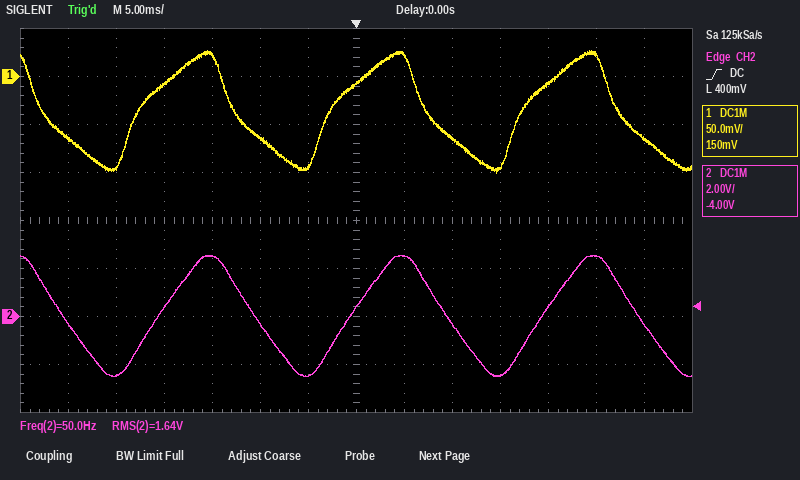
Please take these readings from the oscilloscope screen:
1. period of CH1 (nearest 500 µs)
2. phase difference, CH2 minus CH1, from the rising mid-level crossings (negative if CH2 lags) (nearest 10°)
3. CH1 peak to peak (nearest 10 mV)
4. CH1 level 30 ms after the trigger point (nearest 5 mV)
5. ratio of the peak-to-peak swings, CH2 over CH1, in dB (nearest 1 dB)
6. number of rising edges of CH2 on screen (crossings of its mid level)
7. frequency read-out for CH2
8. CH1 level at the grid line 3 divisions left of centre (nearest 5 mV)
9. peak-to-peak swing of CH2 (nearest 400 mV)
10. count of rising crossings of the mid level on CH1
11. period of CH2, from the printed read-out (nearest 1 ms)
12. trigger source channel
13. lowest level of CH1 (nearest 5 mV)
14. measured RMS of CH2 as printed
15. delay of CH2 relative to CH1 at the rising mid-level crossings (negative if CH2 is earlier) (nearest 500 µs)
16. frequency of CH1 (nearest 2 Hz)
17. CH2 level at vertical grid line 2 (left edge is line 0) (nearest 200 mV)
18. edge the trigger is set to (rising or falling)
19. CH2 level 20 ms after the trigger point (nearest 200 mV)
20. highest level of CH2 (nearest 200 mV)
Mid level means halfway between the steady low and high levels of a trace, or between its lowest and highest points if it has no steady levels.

20.0 ms
-40°
130 mV
-65 mV
32 dB
3
50.0 Hz
20 mV
5.2 V
3
20 ms
CH2
-100 mV
1.64 V
+2.0 ms
50 Hz
-2.4 V
rising
400 mV
2.6 V
